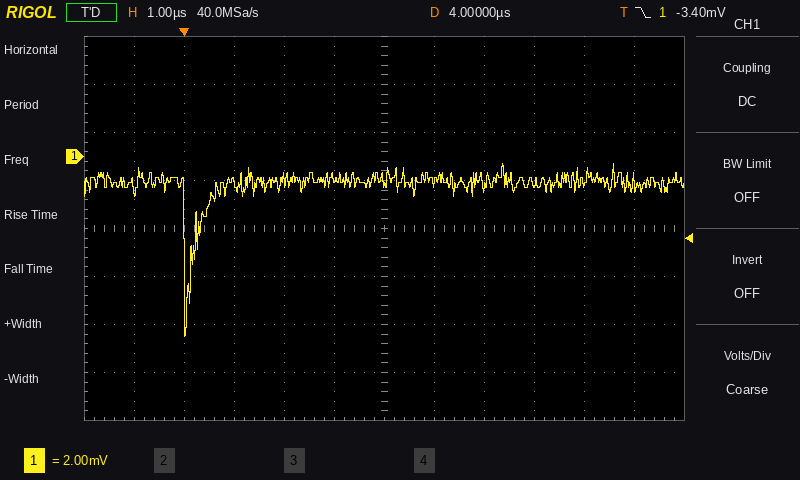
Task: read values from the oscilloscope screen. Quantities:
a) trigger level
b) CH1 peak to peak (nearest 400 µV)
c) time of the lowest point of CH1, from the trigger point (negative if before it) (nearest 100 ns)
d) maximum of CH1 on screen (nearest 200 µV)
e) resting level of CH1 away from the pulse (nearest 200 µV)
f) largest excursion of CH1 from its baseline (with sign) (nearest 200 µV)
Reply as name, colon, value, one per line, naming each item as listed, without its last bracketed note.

trigger level: -3.40 mV
CH1 peak to peak: 7.2 mV
time of the lowest point of CH1, from the trigger point (negative if before it): 0.0 µs
maximum of CH1 on screen: -200 µV
resting level of CH1 away from the pulse: -1.0 mV
largest excursion of CH1 from its baseline (with sign): -6.4 mV
